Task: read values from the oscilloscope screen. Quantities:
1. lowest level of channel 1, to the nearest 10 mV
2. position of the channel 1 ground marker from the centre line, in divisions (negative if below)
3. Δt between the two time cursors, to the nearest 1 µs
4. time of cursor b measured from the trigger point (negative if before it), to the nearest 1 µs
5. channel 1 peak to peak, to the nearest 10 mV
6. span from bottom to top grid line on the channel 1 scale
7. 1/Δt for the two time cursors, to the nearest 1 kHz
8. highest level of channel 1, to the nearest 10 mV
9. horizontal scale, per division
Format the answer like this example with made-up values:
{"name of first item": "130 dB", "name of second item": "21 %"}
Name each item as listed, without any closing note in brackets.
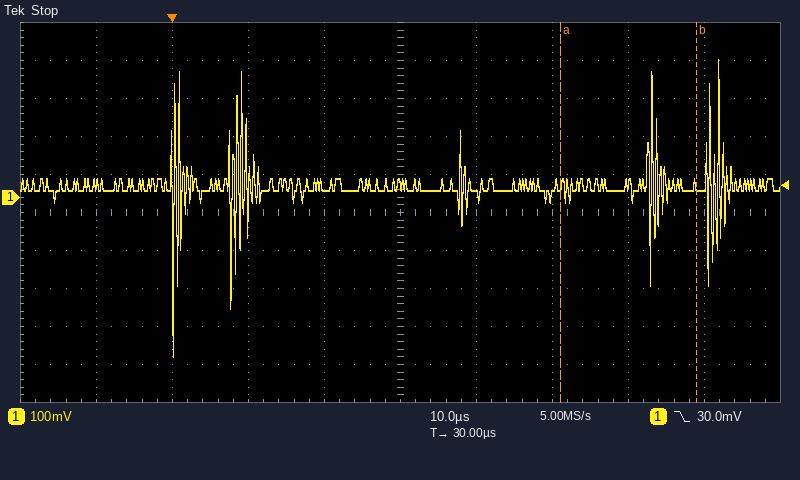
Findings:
{"lowest level of channel 1, to the nearest 10 mV": "-420 mV", "position of the channel 1 ground marker from the centre line, in divisions": "+0.4 div", "Δt between the two time cursors, to the nearest 1 µs": "18 µs", "time of cursor b measured from the trigger point (negative if before it), to the nearest 1 µs": "+69 µs", "channel 1 peak to peak, to the nearest 10 mV": "780 mV", "span from bottom to top grid line on the channel 1 scale": "1 V", "1/Δt for the two time cursors, to the nearest 1 kHz": "56 kHz", "highest level of channel 1, to the nearest 10 mV": "360 mV", "horizontal scale, per division": "10 µs"}
